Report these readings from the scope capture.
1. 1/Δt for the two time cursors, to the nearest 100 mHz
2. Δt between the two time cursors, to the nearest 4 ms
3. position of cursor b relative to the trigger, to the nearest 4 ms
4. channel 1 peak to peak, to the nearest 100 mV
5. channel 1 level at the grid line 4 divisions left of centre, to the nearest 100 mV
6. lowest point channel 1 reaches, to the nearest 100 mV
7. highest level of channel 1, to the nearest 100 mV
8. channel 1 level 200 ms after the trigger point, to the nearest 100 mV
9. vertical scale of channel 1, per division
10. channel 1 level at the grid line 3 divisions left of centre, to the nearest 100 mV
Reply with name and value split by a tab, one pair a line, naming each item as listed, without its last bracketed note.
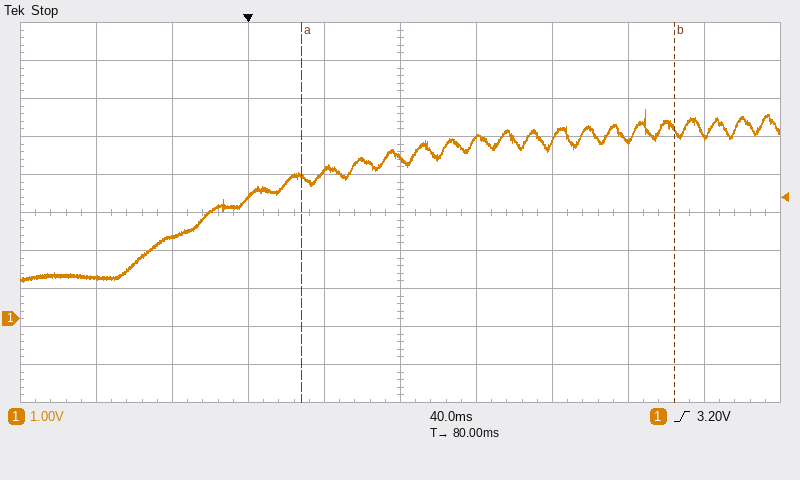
1/Δt for the two time cursors, to the nearest 100 mHz	5.1 Hz
Δt between the two time cursors, to the nearest 4 ms	196 ms
position of cursor b relative to the trigger, to the nearest 4 ms	+224 ms
channel 1 peak to peak, to the nearest 100 mV	4.5 V
channel 1 level at the grid line 4 divisions left of centre, to the nearest 100 mV	1.1 V
lowest point channel 1 reaches, to the nearest 100 mV	1.0 V
highest level of channel 1, to the nearest 100 mV	5.5 V
channel 1 level 200 ms after the trigger point, to the nearest 100 mV	4.7 V
vertical scale of channel 1, per division	1 V
channel 1 level at the grid line 3 divisions left of centre, to the nearest 100 mV	2.2 V
